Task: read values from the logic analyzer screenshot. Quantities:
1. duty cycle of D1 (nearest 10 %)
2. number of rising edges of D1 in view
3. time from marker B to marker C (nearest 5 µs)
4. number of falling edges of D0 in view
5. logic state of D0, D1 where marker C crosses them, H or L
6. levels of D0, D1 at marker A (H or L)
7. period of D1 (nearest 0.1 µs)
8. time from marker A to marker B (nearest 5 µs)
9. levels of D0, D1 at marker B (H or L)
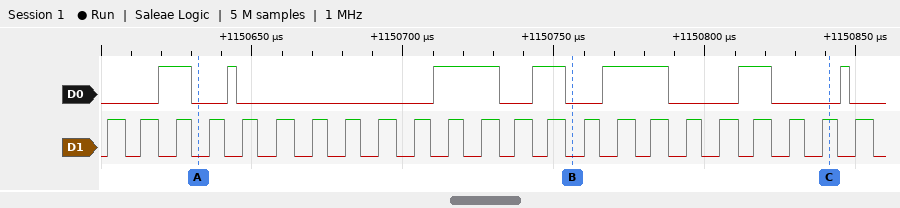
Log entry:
50 %
23
85 µs
7
D0=L, D1=H
D0=L, D1=L
11.3 µs
125 µs
D0=L, D1=L
